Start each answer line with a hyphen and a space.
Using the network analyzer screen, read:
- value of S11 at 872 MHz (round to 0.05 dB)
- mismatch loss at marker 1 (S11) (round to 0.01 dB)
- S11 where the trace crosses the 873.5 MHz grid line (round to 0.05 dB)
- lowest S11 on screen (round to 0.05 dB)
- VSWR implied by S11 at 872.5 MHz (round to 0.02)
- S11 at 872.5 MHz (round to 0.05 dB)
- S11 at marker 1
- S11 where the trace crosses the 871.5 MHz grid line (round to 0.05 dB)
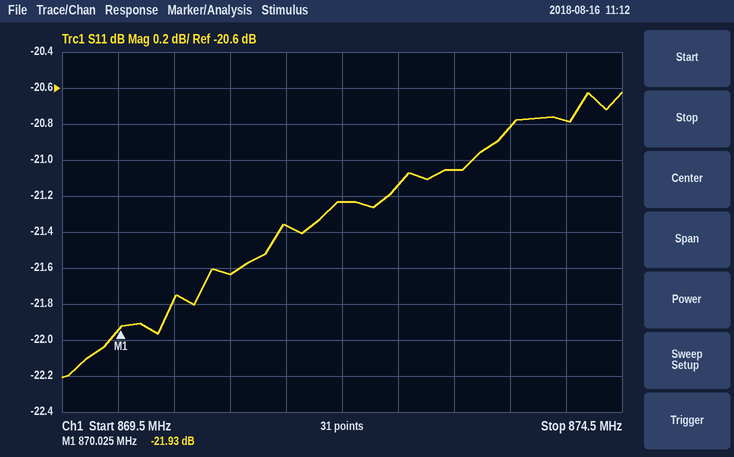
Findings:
- -21.25 dB
- 0.03 dB
- -20.80 dB
- -22.20 dB
- 1.20
- -21.15 dB
- -21.93 dB
- -21.35 dB
